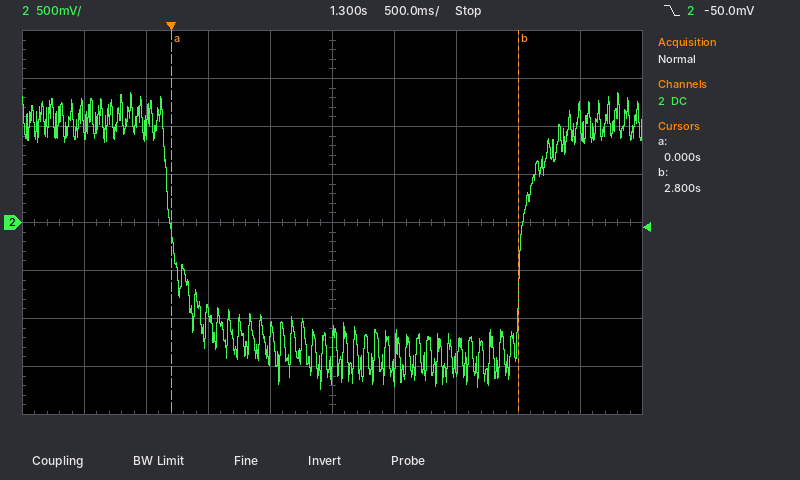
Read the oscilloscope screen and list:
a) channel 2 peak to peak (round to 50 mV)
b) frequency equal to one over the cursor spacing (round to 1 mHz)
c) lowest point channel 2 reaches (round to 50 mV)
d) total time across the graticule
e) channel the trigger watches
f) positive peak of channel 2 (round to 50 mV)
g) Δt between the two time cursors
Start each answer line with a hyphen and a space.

- 3.10 V
- 357 mHz
- -1.75 V
- 5 s
- channel 2
- 1.35 V
- 2.80 s
